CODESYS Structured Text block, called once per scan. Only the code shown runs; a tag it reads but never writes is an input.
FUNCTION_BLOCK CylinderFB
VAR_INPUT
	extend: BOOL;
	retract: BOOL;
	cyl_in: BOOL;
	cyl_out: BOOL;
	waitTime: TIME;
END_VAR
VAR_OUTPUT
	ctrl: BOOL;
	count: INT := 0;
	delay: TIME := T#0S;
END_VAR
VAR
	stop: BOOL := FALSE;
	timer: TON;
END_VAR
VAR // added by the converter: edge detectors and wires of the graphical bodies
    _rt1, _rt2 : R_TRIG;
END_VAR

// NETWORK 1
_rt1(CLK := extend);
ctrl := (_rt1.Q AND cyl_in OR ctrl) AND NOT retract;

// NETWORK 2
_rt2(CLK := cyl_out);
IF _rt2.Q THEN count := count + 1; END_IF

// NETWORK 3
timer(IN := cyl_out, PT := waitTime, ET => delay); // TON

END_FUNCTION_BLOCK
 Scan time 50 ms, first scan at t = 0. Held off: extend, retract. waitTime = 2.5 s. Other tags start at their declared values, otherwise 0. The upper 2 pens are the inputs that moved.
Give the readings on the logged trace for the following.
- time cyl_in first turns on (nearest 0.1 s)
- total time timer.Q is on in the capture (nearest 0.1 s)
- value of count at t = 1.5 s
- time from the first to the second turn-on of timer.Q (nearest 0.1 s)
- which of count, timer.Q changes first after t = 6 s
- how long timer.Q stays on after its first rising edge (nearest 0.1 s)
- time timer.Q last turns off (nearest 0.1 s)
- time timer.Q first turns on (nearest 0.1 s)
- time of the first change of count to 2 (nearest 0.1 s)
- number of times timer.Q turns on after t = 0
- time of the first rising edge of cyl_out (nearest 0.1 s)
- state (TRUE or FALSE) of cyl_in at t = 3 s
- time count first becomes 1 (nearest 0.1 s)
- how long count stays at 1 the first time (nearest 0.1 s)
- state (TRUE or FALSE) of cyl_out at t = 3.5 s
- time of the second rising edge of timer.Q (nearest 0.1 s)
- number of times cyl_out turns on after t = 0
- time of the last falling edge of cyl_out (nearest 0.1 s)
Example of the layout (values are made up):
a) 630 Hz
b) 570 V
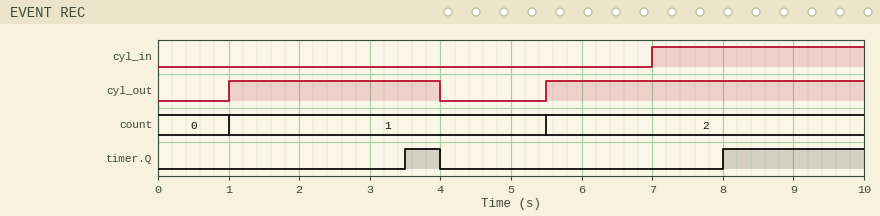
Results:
a) 7.0 s
b) 2.5 s
c) 1
d) 4.5 s
e) timer.Q
f) 0.5 s
g) 4.0 s
h) 3.5 s
i) 5.5 s
j) 2
k) 1.0 s
l) FALSE
m) 1.0 s
n) 4.5 s
o) TRUE
p) 8.0 s
q) 2
r) 4.0 s
